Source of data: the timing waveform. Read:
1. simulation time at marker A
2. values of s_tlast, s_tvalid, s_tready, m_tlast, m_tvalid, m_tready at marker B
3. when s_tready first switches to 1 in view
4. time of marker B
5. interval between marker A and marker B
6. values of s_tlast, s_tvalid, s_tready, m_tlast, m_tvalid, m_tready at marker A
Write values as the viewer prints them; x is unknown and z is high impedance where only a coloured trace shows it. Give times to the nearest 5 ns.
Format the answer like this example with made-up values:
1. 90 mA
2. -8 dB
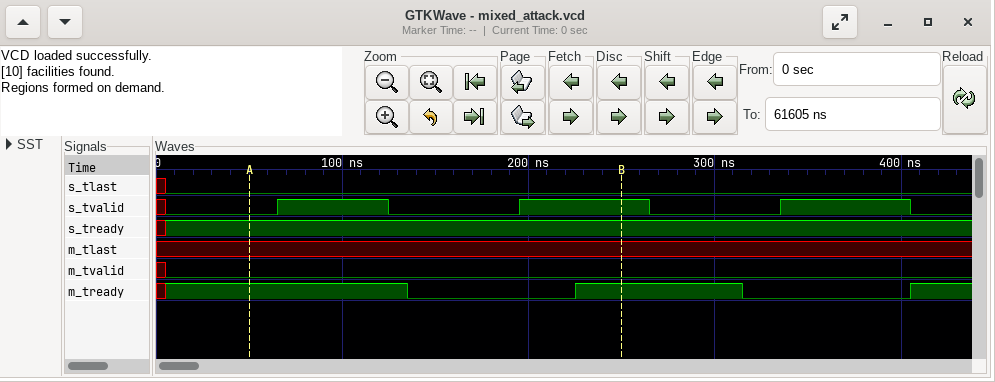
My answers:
1. 50 ns
2. s_tlast=0, s_tvalid=1, s_tready=1, m_tlast=x, m_tvalid=0, m_tready=1
3. 5 ns
4. 250 ns
5. 200 ns
6. s_tlast=0, s_tvalid=0, s_tready=1, m_tlast=x, m_tvalid=0, m_tready=1
